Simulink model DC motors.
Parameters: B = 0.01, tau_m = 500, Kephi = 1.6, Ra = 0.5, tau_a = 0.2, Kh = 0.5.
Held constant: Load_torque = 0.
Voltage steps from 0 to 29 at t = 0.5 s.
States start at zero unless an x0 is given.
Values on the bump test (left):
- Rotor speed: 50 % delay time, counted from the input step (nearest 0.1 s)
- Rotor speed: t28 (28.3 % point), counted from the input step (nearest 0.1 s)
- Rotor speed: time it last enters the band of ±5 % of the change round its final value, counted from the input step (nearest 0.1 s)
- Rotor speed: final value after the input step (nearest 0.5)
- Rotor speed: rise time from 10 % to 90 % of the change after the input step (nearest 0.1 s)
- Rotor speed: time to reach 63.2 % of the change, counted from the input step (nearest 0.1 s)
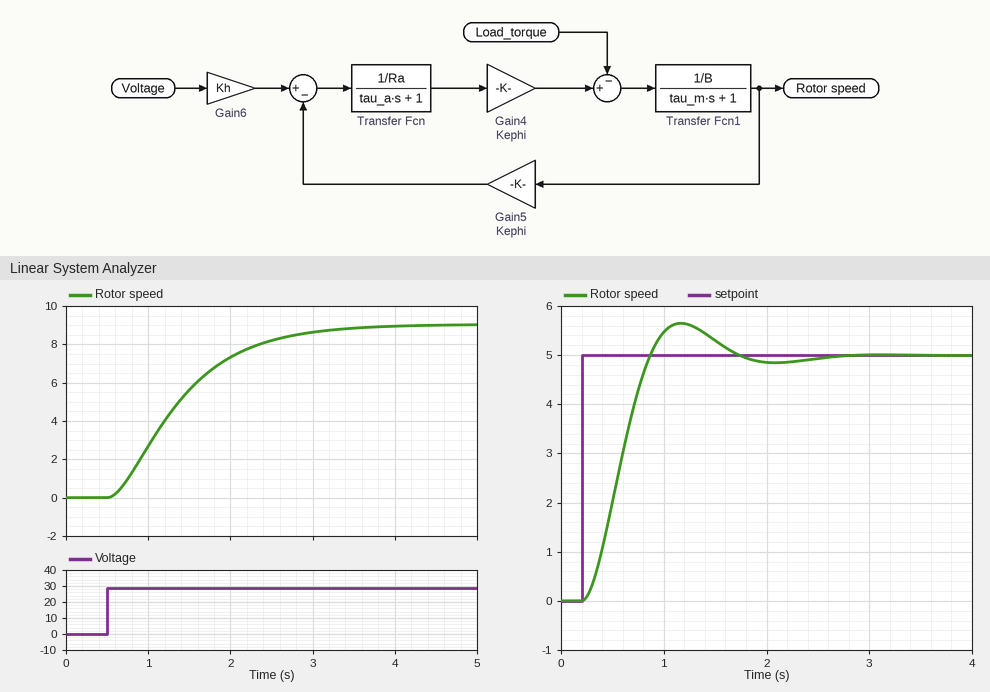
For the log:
0.8 s
0.5 s
2.4 s
9.0
1.7 s
1.0 s
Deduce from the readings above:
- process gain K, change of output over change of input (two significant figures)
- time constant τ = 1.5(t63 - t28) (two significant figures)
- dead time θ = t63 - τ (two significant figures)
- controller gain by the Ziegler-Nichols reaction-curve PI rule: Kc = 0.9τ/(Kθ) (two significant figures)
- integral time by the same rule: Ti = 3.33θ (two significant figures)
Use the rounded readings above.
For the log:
0.31
0.75 s
0.25 s
8.7
0.83 s
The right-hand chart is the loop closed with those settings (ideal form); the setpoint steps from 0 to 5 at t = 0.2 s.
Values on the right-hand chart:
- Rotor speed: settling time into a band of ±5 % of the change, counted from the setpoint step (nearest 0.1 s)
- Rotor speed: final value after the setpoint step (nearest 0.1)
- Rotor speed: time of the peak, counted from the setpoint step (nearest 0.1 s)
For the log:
1.3 s
5.0
1.0 s
